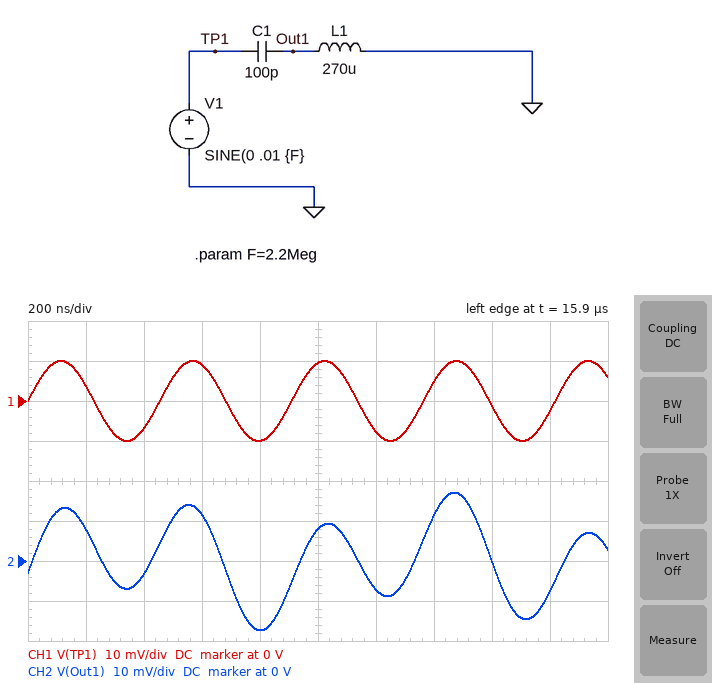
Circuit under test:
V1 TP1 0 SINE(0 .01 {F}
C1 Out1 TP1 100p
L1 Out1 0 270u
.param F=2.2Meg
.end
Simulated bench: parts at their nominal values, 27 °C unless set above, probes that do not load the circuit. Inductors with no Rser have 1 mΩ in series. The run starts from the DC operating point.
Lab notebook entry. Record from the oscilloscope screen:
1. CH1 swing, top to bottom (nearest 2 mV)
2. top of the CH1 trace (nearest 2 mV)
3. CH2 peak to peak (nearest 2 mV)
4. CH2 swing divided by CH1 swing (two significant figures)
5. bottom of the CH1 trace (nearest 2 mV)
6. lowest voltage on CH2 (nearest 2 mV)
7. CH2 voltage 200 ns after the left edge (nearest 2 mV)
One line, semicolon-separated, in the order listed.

20 mV; 10 mV; 34 mV; 1.7; -10 mV; -18 mV; 8 mV
